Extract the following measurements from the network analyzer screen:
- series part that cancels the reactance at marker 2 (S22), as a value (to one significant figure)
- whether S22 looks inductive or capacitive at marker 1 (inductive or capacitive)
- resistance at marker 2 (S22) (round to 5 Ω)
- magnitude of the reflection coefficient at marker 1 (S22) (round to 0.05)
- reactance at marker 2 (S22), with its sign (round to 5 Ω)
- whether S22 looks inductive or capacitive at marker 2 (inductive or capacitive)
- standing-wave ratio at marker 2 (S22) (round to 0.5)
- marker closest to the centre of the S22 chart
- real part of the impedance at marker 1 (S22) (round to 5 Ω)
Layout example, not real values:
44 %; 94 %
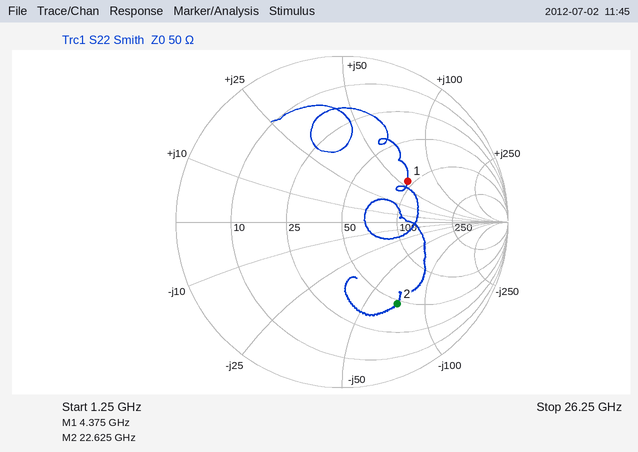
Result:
500 pH; inductive; 45 Ω; 0.45; -70 Ω; capacitive; 4.0; marker 1; 90 Ω
